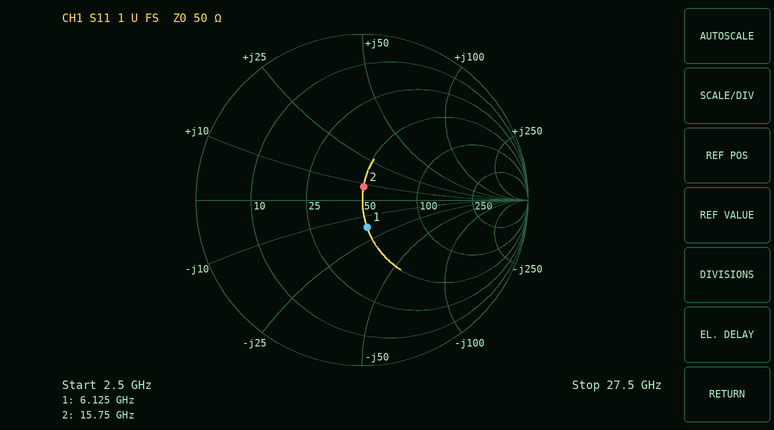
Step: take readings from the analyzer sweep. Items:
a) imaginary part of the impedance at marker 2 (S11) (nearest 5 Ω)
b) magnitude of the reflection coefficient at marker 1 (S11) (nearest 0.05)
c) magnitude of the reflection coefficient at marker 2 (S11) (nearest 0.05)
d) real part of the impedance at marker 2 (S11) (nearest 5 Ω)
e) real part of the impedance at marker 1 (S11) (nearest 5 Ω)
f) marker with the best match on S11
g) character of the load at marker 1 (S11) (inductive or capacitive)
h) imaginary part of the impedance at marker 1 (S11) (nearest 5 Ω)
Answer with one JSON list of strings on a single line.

["+10 Ω", "0.15", "0.10", "50 Ω", "50 Ω", "marker 2", "capacitive", "-15 Ω"]
